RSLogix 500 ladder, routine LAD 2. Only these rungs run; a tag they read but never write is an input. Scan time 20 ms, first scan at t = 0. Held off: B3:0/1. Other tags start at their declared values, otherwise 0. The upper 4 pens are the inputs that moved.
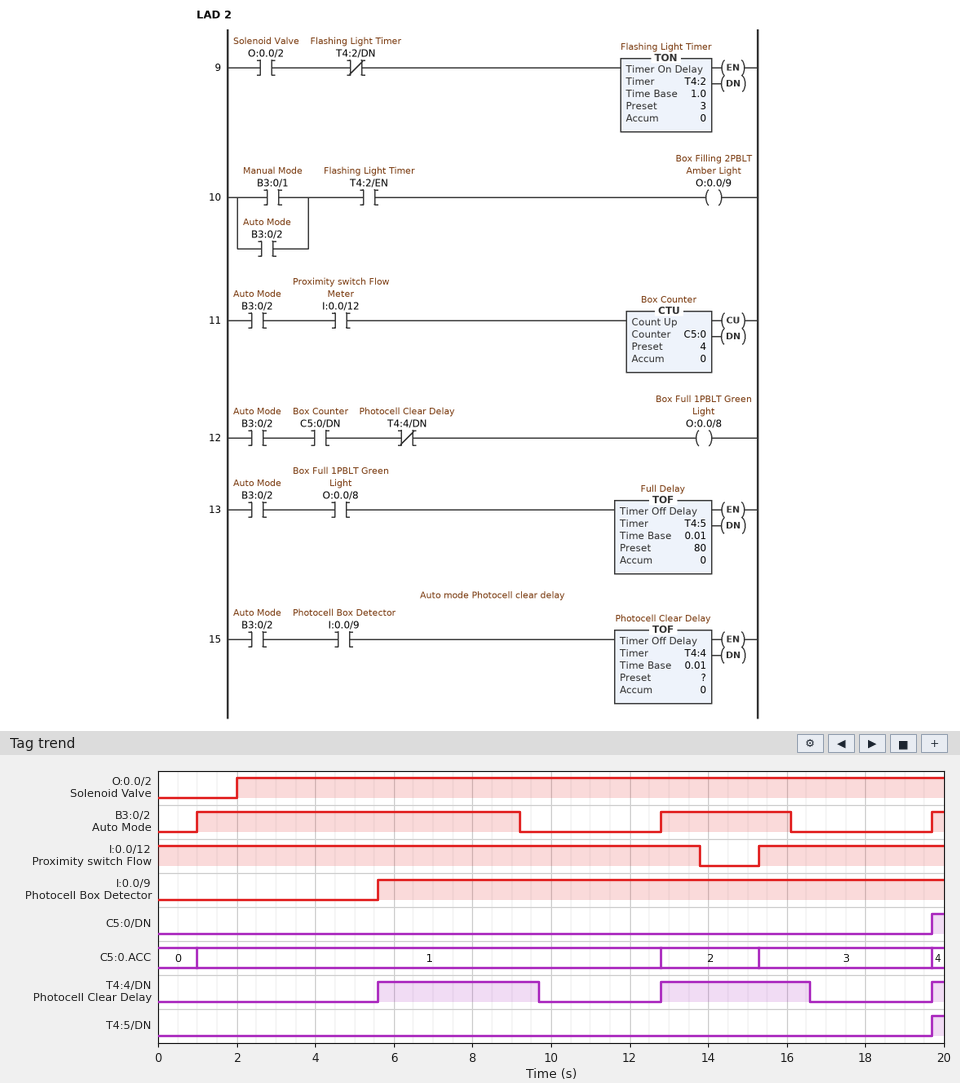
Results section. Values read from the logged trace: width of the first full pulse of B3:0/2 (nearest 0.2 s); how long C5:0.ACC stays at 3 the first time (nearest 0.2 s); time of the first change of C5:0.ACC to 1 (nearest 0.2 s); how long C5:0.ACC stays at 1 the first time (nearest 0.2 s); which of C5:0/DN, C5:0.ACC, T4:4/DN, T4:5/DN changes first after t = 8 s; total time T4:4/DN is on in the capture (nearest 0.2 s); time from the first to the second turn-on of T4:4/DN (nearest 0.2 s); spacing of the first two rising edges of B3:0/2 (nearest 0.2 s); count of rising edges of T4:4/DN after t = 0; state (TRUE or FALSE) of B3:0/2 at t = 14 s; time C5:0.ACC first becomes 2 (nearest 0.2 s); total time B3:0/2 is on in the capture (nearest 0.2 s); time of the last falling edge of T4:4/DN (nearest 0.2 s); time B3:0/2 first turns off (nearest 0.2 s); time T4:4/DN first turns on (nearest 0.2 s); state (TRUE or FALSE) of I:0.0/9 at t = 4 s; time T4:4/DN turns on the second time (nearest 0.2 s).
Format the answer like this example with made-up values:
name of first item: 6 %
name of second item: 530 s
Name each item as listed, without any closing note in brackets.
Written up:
width of the first full pulse of B3:0/2: 8.2 s
how long C5:0.ACC stays at 3 the first time: 4.4 s
time of the first change of C5:0.ACC to 1: 1.0 s
how long C5:0.ACC stays at 1 the first time: 11.8 s
which of C5:0/DN, C5:0.ACC, T4:4/DN, T4:5/DN changes first after t = 8 s: T4:4/DN
total time T4:4/DN is on in the capture: 8.2 s
time from the first to the second turn-on of T4:4/DN: 7.2 s
spacing of the first two rising edges of B3:0/2: 11.8 s
count of rising edges of T4:4/DN after t = 0: 3
state (TRUE or FALSE) of B3:0/2 at t = 14 s: TRUE
time C5:0.ACC first becomes 2: 12.8 s
total time B3:0/2 is on in the capture: 11.8 s
time of the last falling edge of T4:4/DN: 16.6 s
time B3:0/2 first turns off: 9.2 s
time T4:4/DN first turns on: 5.6 s
state (TRUE or FALSE) of I:0.0/9 at t = 4 s: FALSE
time T4:4/DN turns on the second time: 12.8 s
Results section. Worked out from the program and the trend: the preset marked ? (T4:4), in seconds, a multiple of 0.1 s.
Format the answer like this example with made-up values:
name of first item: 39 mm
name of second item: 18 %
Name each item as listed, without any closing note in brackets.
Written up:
the preset marked ? (T4:4), in seconds, a multiple of 0.1 s: 0.5 s
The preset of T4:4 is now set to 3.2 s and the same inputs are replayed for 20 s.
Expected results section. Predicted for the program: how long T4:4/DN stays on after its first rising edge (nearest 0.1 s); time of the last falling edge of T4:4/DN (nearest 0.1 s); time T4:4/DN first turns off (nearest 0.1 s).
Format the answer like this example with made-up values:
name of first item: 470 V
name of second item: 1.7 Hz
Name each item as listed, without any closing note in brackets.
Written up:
how long T4:4/DN stays on after its first rising edge: 6.8 s
time of the last falling edge of T4:4/DN: 19.3 s
time T4:4/DN first turns off: 12.4 s
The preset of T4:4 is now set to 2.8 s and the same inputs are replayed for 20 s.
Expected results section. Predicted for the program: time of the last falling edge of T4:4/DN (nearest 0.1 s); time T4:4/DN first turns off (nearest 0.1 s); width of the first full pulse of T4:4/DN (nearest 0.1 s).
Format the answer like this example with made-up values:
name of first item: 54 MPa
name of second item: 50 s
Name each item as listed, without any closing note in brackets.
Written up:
time of the last falling edge of T4:4/DN: 18.9 s
time T4:4/DN first turns off: 12.0 s
width of the first full pulse of T4:4/DN: 6.4 s
